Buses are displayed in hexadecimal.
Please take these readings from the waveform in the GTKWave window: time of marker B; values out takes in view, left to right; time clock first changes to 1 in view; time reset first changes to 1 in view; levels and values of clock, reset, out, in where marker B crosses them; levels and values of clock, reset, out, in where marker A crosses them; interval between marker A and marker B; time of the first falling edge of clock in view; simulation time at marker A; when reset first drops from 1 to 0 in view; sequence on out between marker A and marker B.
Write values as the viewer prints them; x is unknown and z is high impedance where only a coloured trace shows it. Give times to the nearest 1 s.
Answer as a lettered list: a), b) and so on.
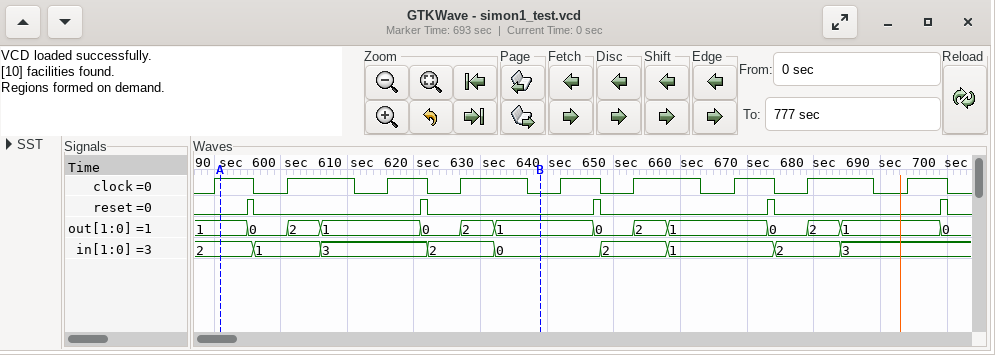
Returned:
a) 639 s
b) 1, 0, 2, 1, 0, 2, 1, 0, 2, 1, 0, 2, 1, 0
c) 590 s
d) 595 s
e) clock=0, reset=0, out=1, in=0
f) clock=1, reset=0, out=1, in=2
g) 48 s
h) 596 s
i) 591 s
j) 596 s
k) 1, 0, 2, 1, 0, 2, 1
